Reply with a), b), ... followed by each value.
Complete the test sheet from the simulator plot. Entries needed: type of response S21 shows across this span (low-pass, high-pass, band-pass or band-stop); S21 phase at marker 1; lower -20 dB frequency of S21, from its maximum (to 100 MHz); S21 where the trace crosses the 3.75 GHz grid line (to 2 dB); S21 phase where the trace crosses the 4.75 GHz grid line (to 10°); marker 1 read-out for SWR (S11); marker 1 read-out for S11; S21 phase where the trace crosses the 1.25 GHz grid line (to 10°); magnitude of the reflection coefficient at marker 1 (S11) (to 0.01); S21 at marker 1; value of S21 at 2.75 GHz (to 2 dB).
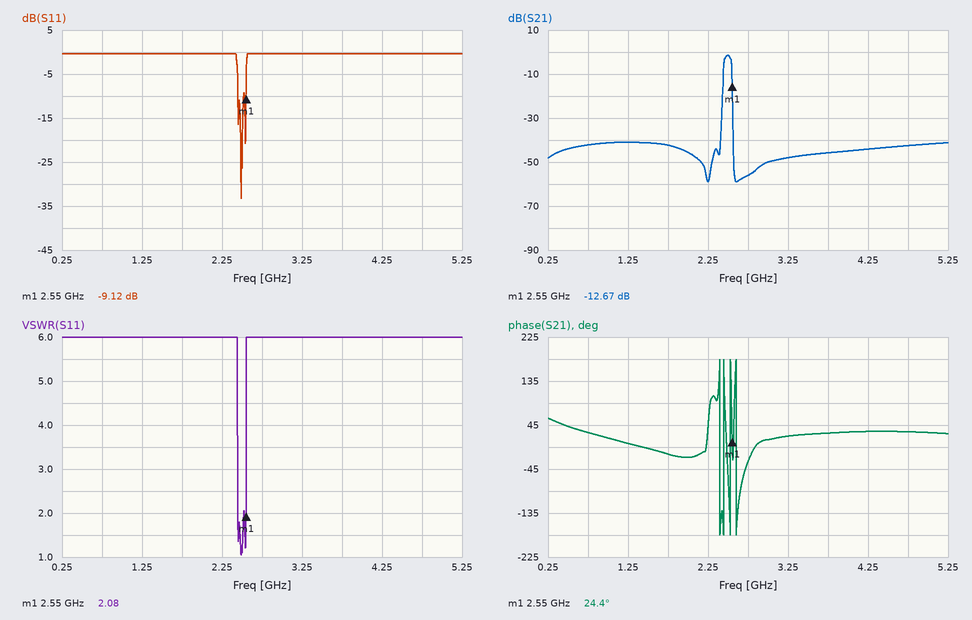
a) band-pass
b) 24.4°
c) 2.4 GHz
d) -46 dB
e) 30°
f) 2.08
g) -9.12 dB
h) 10°
i) 0.35
j) -12.67 dB
k) -56 dB
